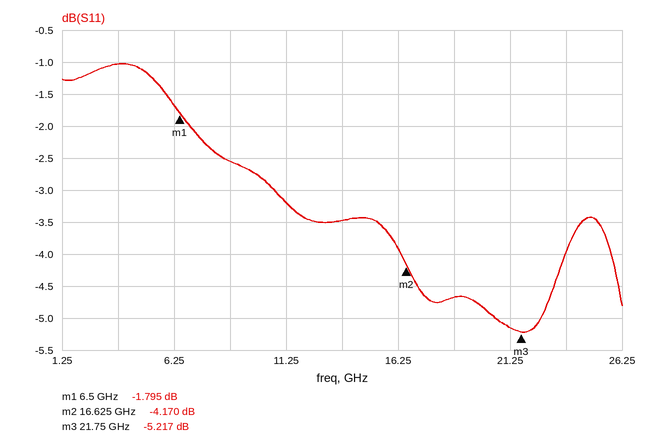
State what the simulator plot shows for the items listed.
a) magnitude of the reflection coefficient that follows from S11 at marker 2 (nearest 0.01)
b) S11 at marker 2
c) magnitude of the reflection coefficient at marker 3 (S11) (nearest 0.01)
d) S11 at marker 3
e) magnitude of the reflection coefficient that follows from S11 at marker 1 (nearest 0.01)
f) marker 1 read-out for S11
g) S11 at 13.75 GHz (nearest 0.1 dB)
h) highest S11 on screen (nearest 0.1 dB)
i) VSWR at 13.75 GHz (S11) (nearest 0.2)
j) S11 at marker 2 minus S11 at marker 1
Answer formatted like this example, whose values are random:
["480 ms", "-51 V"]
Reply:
["0.62", "-4.170 dB", "0.55", "-5.217 dB", "0.81", "-1.795 dB", "-3.5 dB", "-1.0 dB", "5.0", "-2.375 dB"]
